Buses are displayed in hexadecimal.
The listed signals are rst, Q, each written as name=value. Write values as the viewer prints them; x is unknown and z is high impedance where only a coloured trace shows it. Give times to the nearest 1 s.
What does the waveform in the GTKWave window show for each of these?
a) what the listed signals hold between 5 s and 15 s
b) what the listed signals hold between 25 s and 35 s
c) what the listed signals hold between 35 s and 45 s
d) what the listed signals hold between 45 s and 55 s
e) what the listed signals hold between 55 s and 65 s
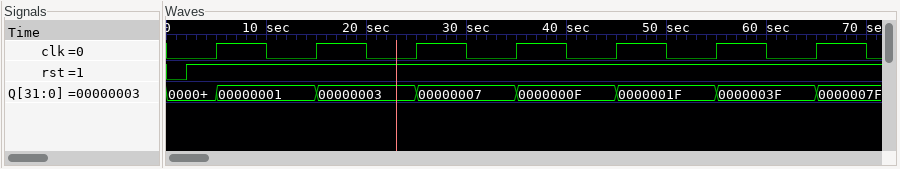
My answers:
rst=1, Q=00000001
rst=1, Q=00000007
rst=1, Q=0000000F
rst=1, Q=0000001F
rst=1, Q=0000003F
